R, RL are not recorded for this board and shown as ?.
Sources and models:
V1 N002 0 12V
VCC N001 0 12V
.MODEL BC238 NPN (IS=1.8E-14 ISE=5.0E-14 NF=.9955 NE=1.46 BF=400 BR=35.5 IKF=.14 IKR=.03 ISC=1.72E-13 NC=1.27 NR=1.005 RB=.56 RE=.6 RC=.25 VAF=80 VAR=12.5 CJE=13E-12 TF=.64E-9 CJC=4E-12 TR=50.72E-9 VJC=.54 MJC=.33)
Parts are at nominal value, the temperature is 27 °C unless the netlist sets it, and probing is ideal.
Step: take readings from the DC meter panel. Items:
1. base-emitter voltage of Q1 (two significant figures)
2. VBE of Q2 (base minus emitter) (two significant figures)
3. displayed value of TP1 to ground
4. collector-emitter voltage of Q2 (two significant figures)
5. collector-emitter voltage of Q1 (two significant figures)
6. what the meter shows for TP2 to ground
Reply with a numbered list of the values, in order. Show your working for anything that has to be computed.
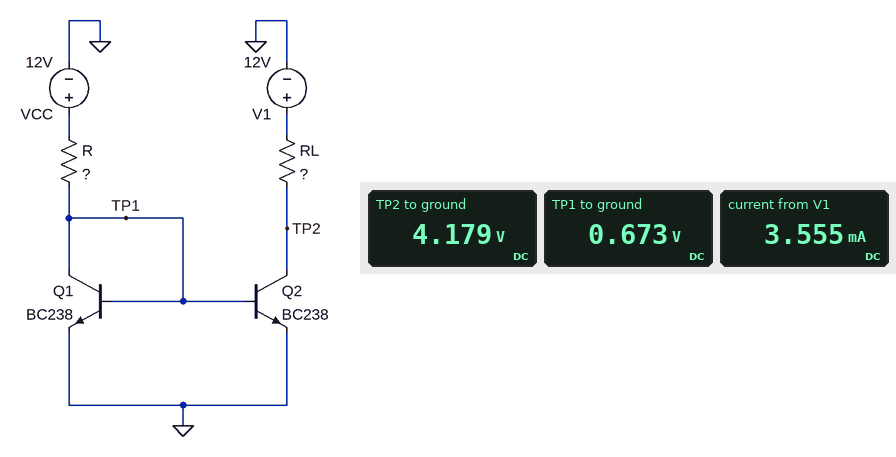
1. 673 mV = 670 mV
2. 673 mV = 670 mV
3. 0.673 V
4. 4.179 V = 4.2 V
5. 673 mV = 670 mV
6. 4.179 V
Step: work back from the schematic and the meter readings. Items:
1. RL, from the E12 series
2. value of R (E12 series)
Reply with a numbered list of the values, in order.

1. 2.2 kΩ
2. 3.3 kΩ
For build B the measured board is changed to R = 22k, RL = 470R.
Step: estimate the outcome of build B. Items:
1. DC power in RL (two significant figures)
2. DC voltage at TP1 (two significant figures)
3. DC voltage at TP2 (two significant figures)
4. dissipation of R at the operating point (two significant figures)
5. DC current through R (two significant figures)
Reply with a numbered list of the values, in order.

1. 160 µW
2. 620 mV
3. 12 V
4. 5.9 mW
5. 520 µA
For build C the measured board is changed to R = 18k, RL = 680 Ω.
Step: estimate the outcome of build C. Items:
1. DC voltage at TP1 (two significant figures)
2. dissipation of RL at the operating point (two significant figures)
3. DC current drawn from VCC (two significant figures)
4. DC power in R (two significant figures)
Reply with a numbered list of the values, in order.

1. 630 mV
2. 350 µW
3. 630 µA
4. 7.2 mW
